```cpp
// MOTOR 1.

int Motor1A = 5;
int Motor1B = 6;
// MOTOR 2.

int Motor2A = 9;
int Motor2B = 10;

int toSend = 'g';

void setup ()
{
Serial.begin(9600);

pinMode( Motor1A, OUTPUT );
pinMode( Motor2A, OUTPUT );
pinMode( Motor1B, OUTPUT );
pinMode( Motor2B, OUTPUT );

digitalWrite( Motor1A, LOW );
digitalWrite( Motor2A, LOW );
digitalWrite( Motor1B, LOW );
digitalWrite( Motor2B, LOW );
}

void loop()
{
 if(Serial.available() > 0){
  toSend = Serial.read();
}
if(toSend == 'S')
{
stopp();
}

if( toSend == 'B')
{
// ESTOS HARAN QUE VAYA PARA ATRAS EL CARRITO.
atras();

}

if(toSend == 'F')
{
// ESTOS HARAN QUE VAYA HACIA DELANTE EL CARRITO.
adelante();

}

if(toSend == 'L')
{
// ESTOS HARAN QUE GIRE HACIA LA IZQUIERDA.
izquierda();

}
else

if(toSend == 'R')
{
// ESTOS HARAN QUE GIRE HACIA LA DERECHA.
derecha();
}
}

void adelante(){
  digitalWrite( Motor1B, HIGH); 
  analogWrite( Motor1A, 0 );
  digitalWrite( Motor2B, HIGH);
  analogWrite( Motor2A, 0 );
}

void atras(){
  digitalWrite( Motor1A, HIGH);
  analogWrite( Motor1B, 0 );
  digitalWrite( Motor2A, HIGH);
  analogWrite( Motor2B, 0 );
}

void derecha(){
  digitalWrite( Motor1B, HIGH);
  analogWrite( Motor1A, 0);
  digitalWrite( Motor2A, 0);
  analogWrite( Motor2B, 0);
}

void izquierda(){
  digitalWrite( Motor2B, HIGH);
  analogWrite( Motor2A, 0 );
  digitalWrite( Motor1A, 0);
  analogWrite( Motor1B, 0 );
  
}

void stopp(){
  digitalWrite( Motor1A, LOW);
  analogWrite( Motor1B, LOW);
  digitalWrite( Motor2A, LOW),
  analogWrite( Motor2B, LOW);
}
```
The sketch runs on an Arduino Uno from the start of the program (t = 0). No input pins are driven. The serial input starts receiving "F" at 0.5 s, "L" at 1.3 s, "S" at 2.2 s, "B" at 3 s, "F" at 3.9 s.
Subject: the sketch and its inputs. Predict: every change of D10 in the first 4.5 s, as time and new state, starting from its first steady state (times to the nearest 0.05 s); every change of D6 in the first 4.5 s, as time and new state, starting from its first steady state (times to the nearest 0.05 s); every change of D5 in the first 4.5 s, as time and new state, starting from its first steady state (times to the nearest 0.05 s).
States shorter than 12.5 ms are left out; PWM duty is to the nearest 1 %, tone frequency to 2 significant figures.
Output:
0 s low; 0.5 s high; 2.2 s low; 3.9 s high
0 s low; 0.5 s high; 1.3 s low; 3.9 s high
0 s low; 3 s high; 3.9 s low
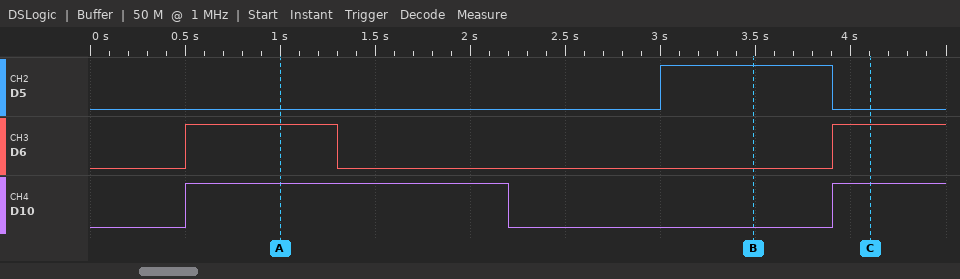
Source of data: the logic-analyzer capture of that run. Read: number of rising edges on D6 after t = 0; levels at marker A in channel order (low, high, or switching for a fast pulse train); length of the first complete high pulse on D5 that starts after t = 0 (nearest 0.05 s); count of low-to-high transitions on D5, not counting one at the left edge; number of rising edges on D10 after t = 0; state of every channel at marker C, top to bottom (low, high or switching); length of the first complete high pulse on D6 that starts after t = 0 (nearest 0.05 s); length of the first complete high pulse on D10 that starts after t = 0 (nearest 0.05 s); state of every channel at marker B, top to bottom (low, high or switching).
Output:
2
D5 low, D6 high, D10 high
0.90 s
1
2
D5 low, D6 high, D10 high
0.80 s
1.70 s
D5 high, D6 low, D10 low
